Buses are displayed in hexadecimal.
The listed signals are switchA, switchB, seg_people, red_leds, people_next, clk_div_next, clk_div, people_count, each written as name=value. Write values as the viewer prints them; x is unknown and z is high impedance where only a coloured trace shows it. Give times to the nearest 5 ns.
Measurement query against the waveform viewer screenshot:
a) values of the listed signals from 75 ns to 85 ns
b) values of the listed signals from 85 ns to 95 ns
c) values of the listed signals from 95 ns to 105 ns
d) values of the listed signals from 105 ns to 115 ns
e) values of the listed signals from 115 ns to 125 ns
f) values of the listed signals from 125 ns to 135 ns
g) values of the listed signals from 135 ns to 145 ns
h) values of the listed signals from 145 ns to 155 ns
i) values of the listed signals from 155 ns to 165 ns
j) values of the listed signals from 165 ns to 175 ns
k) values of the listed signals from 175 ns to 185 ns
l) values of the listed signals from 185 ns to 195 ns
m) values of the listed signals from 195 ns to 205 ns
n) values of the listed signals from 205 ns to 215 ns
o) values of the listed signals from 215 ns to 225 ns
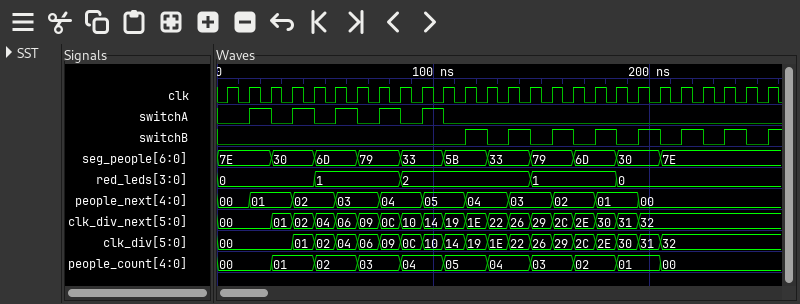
switchA=1, switchB=0, seg_people=79, red_leds=1, people_next=04, clk_div_next=0C, clk_div=09, people_count=03
switchA=0, switchB=0, seg_people=33, red_leds=2, people_next=04, clk_div_next=10, clk_div=0C, people_count=04
switchA=1, switchB=0, seg_people=33, red_leds=2, people_next=05, clk_div_next=14, clk_div=10, people_count=04
switchA=0, switchB=0, seg_people=5B, red_leds=2, people_next=05, clk_div_next=19, clk_div=14, people_count=05
switchA=0, switchB=1, seg_people=5B, red_leds=2, people_next=04, clk_div_next=1E, clk_div=19, people_count=05
switchA=0, switchB=0, seg_people=33, red_leds=2, people_next=04, clk_div_next=22, clk_div=1E, people_count=04
switchA=0, switchB=1, seg_people=33, red_leds=2, people_next=03, clk_div_next=26, clk_div=22, people_count=04
switchA=0, switchB=0, seg_people=79, red_leds=1, people_next=03, clk_div_next=29, clk_div=26, people_count=03
switchA=0, switchB=1, seg_people=79, red_leds=1, people_next=02, clk_div_next=2C, clk_div=29, people_count=03
switchA=0, switchB=0, seg_people=6D, red_leds=1, people_next=02, clk_div_next=2E, clk_div=2C, people_count=02
switchA=0, switchB=1, seg_people=6D, red_leds=1, people_next=01, clk_div_next=30, clk_div=2E, people_count=02
switchA=0, switchB=0, seg_people=30, red_leds=0, people_next=01, clk_div_next=31, clk_div=30, people_count=01
switchA=0, switchB=1, seg_people=30, red_leds=0, people_next=00, clk_div_next=32, clk_div=31, people_count=01
switchA=0, switchB=0, seg_people=7E, red_leds=0, people_next=00, clk_div_next=32, clk_div=32, people_count=00
switchA=0, switchB=1, seg_people=7E, red_leds=0, people_next=00, clk_div_next=32, clk_div=32, people_count=00
